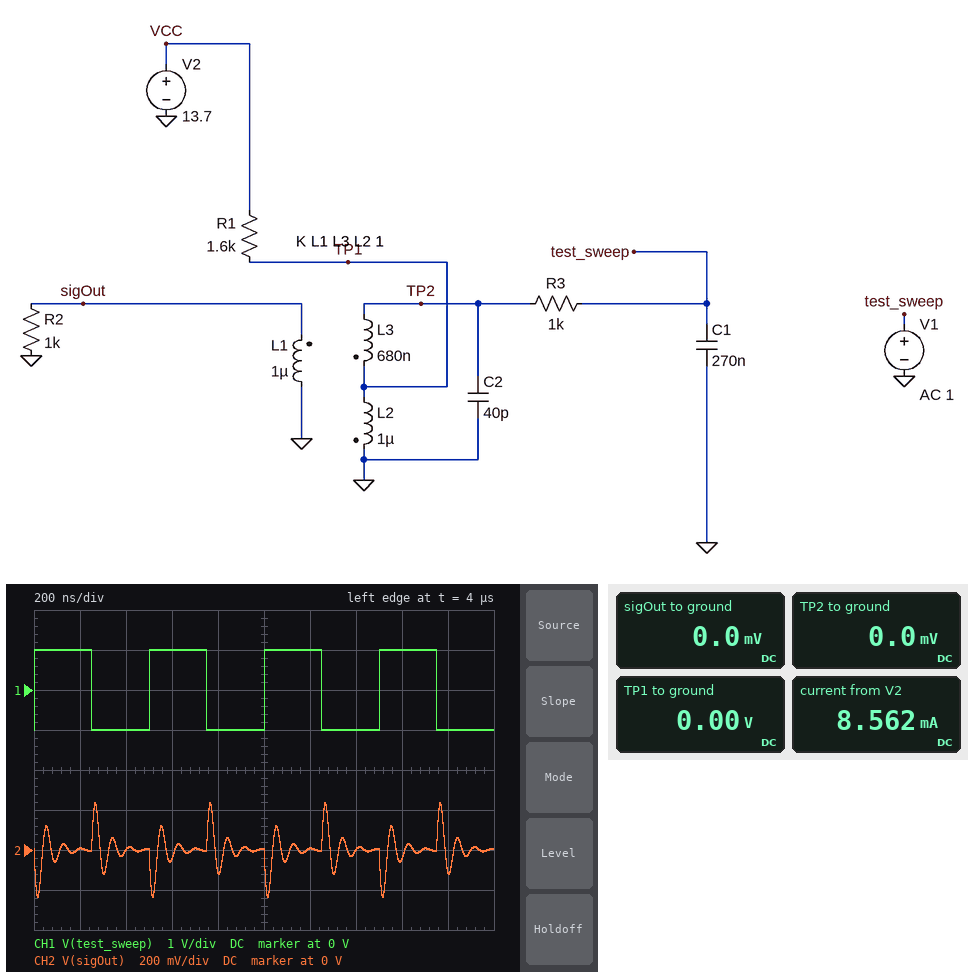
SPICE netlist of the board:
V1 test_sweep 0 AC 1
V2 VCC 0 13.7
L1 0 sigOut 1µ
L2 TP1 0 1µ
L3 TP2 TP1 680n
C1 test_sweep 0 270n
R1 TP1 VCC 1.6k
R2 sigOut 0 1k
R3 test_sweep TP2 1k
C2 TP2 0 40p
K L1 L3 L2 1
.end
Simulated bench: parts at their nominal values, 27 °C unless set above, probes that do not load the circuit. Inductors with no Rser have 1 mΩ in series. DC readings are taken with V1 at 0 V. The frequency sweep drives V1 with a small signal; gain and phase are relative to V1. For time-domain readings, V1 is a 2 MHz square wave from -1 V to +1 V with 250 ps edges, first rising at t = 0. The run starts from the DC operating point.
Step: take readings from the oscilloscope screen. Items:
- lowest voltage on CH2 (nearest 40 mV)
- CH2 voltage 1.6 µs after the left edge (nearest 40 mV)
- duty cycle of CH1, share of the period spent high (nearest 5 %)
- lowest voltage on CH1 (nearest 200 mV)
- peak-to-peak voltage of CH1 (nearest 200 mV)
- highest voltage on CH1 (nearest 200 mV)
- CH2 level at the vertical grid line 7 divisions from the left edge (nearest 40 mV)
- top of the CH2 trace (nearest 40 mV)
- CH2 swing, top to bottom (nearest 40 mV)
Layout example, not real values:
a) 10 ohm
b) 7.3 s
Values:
a) -240 mV
b) -40 mV
c) 50 %
d) -1.0 V
e) 2.0 V
f) 1.0 V
g) 0 V
h) 240 mV
i) 480 mV
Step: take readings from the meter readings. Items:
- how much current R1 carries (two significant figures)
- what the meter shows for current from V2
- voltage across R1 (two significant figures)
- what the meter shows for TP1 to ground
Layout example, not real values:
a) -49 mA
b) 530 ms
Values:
a) 8.6 mA
b) 8.562 mA
c) 14 V
d) 0.00 V
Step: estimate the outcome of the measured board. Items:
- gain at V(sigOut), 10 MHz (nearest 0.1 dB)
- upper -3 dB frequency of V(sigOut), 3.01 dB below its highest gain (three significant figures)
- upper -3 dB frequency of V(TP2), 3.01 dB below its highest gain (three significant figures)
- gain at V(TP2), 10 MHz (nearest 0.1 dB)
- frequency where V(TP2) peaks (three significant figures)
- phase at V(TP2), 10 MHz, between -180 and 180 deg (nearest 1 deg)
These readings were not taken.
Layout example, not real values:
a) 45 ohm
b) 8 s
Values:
a) -13.9 dB
b) 17.1 MHz
c) 17.1 MHz
d) -8.7 dB
e) 13.8 MHz
f) 57 deg
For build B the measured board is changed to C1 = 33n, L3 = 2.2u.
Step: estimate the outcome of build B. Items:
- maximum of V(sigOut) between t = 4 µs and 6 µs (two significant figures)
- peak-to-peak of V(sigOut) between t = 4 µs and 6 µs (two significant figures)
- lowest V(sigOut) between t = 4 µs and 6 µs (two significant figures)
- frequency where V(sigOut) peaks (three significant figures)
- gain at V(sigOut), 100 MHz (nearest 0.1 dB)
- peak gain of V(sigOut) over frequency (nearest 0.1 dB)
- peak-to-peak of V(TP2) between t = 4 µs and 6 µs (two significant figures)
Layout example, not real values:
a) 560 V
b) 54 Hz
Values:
a) 230 mV
b) 460 mV
c) -230 mV
d) 10.1 MHz
e) -35.8 dB
f) -9.9 dB
g) 1.1 V
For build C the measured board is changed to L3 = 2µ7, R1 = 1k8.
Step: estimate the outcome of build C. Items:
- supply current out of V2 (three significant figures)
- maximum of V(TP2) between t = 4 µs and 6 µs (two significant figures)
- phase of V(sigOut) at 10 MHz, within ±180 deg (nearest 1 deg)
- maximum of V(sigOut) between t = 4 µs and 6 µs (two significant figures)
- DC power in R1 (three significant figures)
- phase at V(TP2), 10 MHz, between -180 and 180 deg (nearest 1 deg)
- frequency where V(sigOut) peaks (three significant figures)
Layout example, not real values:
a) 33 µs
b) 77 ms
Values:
a) 7.61 mA
b) 590 mV
c) 169 deg
d) 220 mV
e) 104 mW
f) -11 deg
g) 9.52 MHz
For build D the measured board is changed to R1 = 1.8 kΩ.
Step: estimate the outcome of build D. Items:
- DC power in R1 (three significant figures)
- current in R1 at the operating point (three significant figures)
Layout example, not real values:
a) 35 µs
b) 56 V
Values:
a) 104 mW
b) 7.61 mA
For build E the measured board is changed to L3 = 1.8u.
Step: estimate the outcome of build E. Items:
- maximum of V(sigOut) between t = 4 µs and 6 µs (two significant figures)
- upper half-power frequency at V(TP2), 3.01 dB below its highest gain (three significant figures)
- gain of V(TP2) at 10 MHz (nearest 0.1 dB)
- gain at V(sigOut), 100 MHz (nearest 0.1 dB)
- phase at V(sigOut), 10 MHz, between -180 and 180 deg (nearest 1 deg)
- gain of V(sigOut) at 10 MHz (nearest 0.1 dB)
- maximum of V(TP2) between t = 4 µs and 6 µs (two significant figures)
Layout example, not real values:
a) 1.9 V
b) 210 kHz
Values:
a) 230 mV
b) 13.6 MHz
c) -2.6 dB
d) -35.3 dB
e) -163 deg
f) -10.0 dB
g) 540 mV
